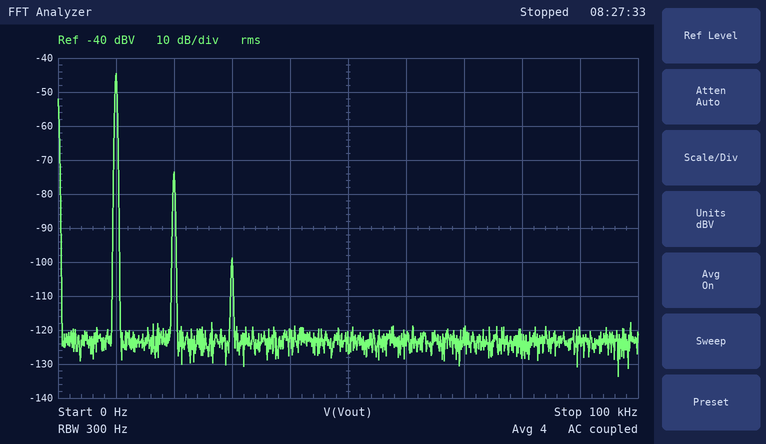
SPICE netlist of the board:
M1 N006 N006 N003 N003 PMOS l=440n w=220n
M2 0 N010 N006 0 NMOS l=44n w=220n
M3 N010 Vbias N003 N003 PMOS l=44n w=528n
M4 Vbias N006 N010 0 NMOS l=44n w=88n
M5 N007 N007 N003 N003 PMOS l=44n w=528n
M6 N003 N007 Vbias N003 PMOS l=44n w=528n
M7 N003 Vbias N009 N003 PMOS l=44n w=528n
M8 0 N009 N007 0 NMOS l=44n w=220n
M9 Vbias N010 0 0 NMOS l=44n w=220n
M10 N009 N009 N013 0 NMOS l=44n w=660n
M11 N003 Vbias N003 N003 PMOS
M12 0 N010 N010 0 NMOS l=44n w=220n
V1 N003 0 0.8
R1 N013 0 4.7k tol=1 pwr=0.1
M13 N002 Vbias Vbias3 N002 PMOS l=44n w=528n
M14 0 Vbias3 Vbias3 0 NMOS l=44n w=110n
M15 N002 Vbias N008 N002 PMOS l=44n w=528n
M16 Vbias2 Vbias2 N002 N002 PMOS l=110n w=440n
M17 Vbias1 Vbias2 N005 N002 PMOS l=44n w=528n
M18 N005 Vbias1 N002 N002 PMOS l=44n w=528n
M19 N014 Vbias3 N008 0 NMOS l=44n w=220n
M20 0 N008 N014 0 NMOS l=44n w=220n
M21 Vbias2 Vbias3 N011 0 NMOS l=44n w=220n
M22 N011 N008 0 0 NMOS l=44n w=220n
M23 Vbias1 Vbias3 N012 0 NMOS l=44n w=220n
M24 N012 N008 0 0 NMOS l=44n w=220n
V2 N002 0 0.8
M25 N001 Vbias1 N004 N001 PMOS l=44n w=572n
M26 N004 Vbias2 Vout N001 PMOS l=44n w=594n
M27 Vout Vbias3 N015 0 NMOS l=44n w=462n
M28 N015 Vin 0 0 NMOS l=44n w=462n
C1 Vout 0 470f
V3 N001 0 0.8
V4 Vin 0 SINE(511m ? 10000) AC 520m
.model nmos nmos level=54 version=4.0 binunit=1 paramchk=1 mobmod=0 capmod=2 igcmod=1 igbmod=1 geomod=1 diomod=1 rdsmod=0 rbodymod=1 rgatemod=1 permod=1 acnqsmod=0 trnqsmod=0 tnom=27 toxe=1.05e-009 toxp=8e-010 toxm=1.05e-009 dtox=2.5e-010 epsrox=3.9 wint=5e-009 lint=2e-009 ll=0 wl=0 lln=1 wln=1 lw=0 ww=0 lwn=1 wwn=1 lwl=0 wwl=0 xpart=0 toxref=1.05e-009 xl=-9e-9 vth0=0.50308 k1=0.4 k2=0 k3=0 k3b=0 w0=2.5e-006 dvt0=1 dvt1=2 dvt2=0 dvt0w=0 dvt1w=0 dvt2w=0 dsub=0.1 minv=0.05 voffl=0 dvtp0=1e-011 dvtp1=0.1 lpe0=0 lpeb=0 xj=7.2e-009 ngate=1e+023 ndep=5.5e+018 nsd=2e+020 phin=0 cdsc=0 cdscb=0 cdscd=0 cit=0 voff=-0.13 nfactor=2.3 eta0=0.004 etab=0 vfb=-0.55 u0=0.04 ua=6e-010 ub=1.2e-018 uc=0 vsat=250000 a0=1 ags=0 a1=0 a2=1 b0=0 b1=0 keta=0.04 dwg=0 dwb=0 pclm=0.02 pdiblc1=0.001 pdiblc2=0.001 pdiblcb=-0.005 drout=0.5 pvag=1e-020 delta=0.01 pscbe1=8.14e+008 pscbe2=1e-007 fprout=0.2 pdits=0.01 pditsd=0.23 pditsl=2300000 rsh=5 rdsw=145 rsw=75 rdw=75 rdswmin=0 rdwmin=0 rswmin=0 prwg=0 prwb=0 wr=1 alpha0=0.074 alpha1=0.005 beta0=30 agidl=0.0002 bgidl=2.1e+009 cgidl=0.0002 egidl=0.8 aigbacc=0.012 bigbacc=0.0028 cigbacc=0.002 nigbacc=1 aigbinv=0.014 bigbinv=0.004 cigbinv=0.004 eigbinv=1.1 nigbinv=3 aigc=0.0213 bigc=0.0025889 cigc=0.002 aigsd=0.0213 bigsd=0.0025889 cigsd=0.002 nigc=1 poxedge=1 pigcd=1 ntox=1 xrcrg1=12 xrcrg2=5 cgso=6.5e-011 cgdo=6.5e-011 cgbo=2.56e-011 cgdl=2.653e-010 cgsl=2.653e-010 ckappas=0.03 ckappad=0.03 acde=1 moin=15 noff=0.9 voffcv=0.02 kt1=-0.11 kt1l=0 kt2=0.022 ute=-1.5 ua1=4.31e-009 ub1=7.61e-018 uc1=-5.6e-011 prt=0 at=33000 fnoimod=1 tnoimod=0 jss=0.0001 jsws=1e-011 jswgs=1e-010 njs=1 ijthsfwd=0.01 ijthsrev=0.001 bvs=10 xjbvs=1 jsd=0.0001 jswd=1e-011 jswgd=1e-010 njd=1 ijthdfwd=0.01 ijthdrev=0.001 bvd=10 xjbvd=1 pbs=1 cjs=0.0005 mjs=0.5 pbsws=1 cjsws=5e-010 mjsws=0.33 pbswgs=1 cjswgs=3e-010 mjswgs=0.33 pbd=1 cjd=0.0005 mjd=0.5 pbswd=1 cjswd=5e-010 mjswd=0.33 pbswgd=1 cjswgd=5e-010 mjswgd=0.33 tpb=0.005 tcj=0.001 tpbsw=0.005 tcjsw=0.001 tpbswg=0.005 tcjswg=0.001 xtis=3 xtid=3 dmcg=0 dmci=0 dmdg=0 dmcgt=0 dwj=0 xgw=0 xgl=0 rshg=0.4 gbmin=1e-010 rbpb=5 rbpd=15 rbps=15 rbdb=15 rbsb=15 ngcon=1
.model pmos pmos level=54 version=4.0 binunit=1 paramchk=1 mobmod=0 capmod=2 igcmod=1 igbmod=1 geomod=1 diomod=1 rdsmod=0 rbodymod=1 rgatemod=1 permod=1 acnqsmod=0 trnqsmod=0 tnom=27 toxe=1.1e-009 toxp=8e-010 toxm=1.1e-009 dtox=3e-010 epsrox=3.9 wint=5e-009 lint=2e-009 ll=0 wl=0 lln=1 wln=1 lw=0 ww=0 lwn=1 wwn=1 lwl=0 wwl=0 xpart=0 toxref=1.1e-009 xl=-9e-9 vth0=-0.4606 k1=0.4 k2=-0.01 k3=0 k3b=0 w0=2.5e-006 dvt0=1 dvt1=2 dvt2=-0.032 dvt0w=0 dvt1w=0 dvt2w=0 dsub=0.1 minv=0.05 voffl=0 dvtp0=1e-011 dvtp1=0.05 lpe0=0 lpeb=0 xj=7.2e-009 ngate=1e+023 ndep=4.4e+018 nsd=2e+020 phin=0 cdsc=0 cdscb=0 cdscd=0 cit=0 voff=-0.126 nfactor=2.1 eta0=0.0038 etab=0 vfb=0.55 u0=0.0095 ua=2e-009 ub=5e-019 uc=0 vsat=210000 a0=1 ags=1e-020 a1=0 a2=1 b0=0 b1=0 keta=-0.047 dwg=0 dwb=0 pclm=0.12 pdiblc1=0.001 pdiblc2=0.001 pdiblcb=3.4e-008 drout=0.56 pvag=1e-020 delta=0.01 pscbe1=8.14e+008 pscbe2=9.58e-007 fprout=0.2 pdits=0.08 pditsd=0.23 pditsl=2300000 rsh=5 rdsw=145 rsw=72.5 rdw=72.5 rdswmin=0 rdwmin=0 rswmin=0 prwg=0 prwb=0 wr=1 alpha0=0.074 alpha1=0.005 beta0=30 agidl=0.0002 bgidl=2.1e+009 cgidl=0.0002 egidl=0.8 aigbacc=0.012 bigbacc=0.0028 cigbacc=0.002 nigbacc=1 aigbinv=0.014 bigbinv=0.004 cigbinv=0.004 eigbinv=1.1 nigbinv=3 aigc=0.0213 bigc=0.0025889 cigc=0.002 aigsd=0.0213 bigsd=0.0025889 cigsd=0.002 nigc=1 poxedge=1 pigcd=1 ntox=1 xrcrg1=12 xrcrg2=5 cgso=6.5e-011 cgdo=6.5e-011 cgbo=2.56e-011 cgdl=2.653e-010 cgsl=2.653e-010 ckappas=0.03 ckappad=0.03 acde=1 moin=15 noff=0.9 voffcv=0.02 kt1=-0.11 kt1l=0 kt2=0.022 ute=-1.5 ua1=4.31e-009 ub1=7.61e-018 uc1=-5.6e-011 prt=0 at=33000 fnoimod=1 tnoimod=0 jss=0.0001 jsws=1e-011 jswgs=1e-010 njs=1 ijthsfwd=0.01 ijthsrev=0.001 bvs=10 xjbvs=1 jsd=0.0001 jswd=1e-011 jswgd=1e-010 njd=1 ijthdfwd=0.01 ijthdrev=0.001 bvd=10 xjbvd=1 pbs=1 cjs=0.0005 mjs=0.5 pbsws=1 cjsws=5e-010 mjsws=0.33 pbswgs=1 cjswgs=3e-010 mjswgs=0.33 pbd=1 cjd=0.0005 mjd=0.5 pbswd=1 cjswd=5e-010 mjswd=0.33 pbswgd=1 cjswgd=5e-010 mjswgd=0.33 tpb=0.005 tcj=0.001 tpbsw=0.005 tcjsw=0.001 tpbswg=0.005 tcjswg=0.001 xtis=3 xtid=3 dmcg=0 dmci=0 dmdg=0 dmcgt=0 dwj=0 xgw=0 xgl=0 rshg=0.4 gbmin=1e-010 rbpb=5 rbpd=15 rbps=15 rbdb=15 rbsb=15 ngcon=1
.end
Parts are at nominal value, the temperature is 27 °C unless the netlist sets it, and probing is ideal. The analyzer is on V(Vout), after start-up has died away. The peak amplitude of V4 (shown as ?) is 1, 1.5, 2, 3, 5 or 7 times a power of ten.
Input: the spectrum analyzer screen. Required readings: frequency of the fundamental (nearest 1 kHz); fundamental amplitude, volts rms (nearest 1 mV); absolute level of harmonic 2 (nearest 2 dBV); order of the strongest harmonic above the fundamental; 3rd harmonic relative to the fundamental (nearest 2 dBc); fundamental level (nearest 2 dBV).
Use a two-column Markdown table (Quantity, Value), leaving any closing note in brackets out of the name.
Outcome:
| Quantity | Value |
|---|---|
| frequency of the fundamental | 10 kHz |
| fundamental amplitude, volts rms | 6 mV |
| absolute level of harmonic 2 | -74 dBV |
| order of the strongest harmonic above the fundamental | 2 |
| 3rd harmonic relative to the fundamental | -54 dBc |
| fundamental level | -44 dBV |
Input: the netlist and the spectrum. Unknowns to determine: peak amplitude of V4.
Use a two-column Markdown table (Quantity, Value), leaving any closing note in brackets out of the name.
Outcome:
| Quantity | Value |
|---|---|
| peak amplitude of V4 | 1 mV |
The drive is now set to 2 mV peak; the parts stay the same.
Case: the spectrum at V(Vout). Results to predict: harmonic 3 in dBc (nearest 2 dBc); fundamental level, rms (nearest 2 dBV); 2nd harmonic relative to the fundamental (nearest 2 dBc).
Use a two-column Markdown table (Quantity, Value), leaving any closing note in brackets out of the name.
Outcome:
| Quantity | Value |
|---|---|
| harmonic 3 in dBc | -42 dBc |
| fundamental level, rms | -38 dBV |
| 2nd harmonic relative to the fundamental | -22 dBc |
